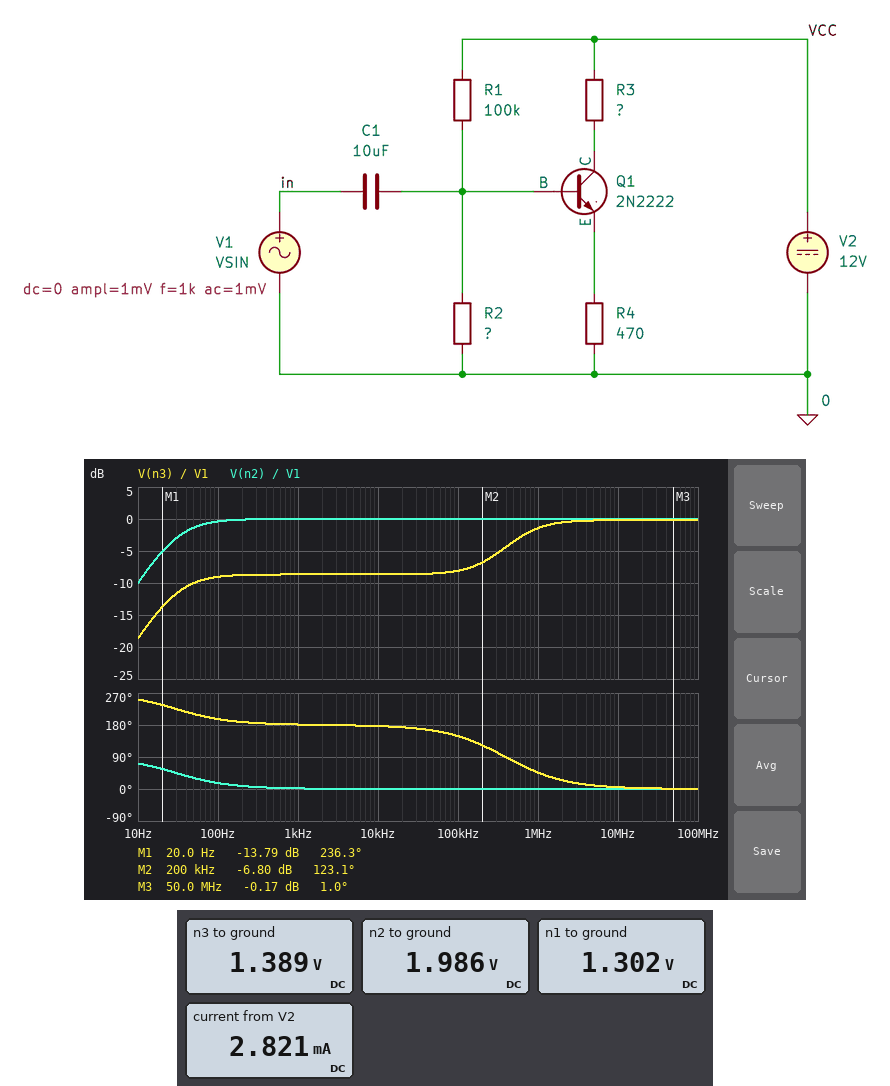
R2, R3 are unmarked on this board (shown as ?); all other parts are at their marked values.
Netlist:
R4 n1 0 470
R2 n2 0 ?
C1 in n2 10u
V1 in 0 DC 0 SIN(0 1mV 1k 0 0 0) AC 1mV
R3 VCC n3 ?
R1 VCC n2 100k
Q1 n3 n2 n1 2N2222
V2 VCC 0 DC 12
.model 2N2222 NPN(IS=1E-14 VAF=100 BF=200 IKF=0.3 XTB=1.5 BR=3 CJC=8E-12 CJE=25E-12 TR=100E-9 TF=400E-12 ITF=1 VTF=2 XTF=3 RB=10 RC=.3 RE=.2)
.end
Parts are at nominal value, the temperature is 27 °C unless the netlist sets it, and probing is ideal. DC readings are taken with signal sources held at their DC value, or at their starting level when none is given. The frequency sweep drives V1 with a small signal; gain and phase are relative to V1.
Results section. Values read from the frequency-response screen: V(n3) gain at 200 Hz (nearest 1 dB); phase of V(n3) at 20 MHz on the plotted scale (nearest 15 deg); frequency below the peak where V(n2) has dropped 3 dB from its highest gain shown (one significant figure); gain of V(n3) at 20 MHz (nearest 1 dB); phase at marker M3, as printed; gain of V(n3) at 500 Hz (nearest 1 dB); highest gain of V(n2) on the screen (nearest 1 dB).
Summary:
-9 dB
0 deg
30 Hz
0 dB
1.0 deg
-9 dB
0 dB
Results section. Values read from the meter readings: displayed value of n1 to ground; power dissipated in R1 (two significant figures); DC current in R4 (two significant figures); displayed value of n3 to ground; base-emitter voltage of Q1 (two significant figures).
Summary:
1.302 V
1.0 mW
2.8 mA
1.389 V
680 mV
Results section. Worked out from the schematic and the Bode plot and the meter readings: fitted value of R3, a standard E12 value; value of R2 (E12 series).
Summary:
3.9 kΩ
39 kΩ
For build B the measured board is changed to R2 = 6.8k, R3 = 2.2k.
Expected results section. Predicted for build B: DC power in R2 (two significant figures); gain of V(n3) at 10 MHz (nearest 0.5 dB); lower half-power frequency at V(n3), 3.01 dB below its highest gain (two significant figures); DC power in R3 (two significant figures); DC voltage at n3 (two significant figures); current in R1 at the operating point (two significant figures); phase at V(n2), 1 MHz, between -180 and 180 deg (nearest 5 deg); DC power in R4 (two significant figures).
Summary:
84 µW
11.0 dB
2.6 Hz
180 µW
11 V
110 µA
0 deg
39 µW
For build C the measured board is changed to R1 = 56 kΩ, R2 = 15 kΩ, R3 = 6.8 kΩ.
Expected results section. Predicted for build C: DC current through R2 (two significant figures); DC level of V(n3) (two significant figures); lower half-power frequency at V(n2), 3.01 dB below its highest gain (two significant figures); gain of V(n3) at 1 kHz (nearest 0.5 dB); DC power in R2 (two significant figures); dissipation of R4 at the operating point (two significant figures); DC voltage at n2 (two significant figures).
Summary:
99 µA
870 mV
32 Hz
-9.0 dB
150 µW
1.4 mW
1.5 V
